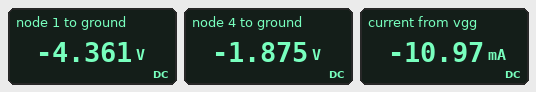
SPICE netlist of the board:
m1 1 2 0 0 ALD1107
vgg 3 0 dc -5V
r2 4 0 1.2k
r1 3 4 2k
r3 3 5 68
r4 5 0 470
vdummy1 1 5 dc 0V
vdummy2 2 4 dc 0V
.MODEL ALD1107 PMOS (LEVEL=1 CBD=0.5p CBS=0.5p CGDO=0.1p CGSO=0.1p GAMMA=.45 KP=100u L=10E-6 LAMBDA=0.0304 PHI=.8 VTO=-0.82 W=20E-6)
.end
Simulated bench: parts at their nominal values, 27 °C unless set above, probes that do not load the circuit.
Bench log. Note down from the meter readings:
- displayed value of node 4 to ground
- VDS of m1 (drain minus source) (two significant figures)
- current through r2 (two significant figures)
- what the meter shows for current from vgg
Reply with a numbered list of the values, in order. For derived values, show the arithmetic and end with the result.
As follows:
1. -1.875 V
2. -4.361 V = -4.4 V
3. (0 V - (-1.875 V)) / 1.2 kΩ = 1.6 mA
4. -10.97 mA
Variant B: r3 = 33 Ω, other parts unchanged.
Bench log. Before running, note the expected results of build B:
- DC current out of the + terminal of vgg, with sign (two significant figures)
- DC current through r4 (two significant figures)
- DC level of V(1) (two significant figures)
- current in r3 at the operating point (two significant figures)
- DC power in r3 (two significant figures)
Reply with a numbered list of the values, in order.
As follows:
1. -12 mA
2. 9.9 mA
3. -4.7 V
4. 10 mA
5. 3.3 mW
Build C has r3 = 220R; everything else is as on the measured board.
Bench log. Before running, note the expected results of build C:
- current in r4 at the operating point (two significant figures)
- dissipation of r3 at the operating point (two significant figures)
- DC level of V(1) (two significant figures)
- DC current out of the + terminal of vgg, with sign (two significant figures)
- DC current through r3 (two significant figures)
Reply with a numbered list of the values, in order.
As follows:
1. 7.2 mA
2. 12 mW
3. -3.4 V
4. -8.9 mA
5. 7.3 mA
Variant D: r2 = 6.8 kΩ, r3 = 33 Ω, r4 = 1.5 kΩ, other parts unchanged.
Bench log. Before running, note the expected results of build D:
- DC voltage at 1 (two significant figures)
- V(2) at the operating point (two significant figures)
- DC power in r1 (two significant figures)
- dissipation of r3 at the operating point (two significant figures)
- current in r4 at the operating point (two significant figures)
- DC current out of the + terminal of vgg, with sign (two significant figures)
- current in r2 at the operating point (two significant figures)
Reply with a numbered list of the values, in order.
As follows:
1. -4.9 V
2. -3.9 V
3. 650 µW
4. 610 µW
5. 3.2 mA
6. -4.9 mA
7. 570 µA
